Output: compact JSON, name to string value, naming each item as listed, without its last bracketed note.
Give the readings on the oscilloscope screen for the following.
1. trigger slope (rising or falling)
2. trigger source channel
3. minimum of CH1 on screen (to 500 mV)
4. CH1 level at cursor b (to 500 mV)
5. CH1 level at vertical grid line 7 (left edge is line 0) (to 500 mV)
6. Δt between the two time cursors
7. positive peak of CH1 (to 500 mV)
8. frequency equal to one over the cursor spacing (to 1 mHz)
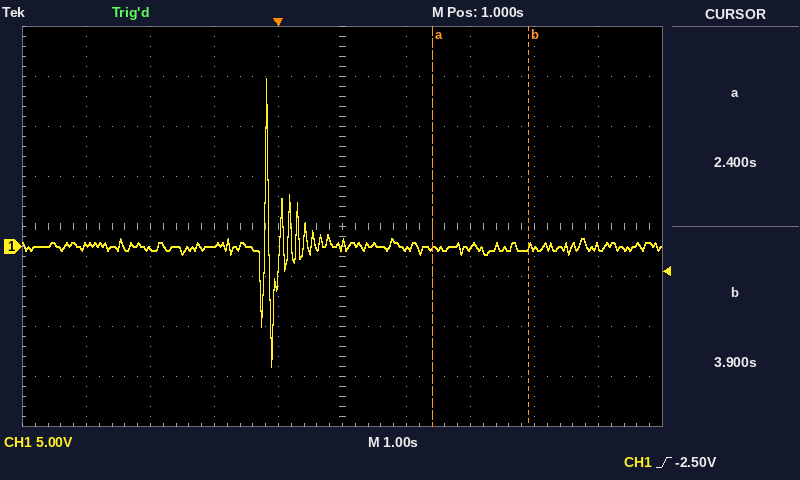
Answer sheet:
{"trigger slope": "rising", "trigger source channel": "CH1", "minimum of CH1 on screen": "-12.0 V", "CH1 level at cursor b": "0.0 V", "CH1 level at vertical grid line 7 (left edge is line 0)": "0.0 V", "Δt between the two time cursors": "1.5 s", "positive peak of CH1": "17.0 V", "frequency equal to one over the cursor spacing": "667 mHz"}
